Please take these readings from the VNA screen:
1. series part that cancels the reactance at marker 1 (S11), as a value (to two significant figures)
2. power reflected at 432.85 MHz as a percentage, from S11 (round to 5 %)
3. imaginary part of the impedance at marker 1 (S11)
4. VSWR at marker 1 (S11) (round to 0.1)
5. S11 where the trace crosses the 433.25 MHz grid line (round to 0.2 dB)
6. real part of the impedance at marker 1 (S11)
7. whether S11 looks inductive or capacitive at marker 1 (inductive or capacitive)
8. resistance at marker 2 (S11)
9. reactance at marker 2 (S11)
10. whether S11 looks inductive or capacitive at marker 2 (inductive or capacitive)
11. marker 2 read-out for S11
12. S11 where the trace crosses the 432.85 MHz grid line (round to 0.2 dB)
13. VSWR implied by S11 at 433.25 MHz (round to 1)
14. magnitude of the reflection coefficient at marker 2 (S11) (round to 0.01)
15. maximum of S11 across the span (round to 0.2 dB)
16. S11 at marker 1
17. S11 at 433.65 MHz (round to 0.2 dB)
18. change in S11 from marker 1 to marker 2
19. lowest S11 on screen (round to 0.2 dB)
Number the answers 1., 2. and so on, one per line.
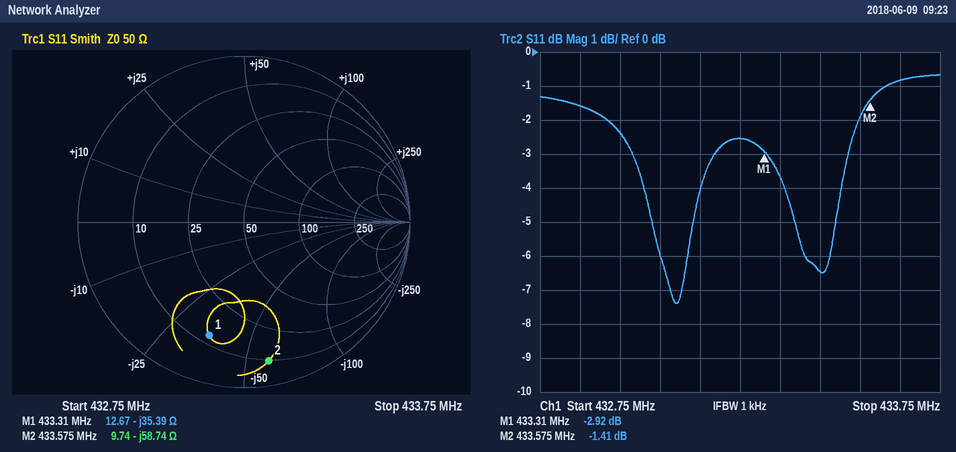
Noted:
1. 13 nH
2. 70 %
3. -35.39 Ω
4. 6.0
5. -2.6 dB
6. 12.67 Ω
7. capacitive
8. 9.74 Ω
9. -58.74 Ω
10. capacitive
11. -1.41 dB
12. -1.6 dB
13. 7
14. 0.85
15. -0.6 dB
16. -2.92 dB
17. -0.8 dB
18. 1.51 dB
19. -7.4 dB
